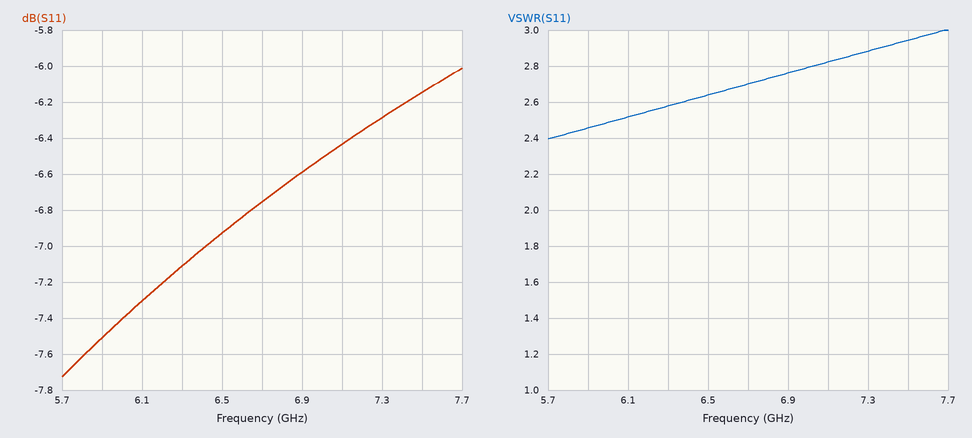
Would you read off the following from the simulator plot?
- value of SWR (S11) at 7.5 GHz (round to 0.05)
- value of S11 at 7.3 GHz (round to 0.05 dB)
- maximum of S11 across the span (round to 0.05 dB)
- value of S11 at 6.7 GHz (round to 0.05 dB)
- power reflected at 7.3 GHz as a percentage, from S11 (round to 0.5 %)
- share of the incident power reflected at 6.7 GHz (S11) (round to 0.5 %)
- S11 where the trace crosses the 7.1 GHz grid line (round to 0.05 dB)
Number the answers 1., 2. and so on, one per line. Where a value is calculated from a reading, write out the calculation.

1. 2.95
2. -6.30 dB
3. -6.00 dB
4. -6.75 dB
5. 10^(-6.3/10) ≈ 23.4 %, so 23.5 % to the nearest 0.5 %
6. 10^(-6.75/10) ≈ 21.1 %, so 21.0 % to the nearest 0.5 %
7. -6.45 dB
